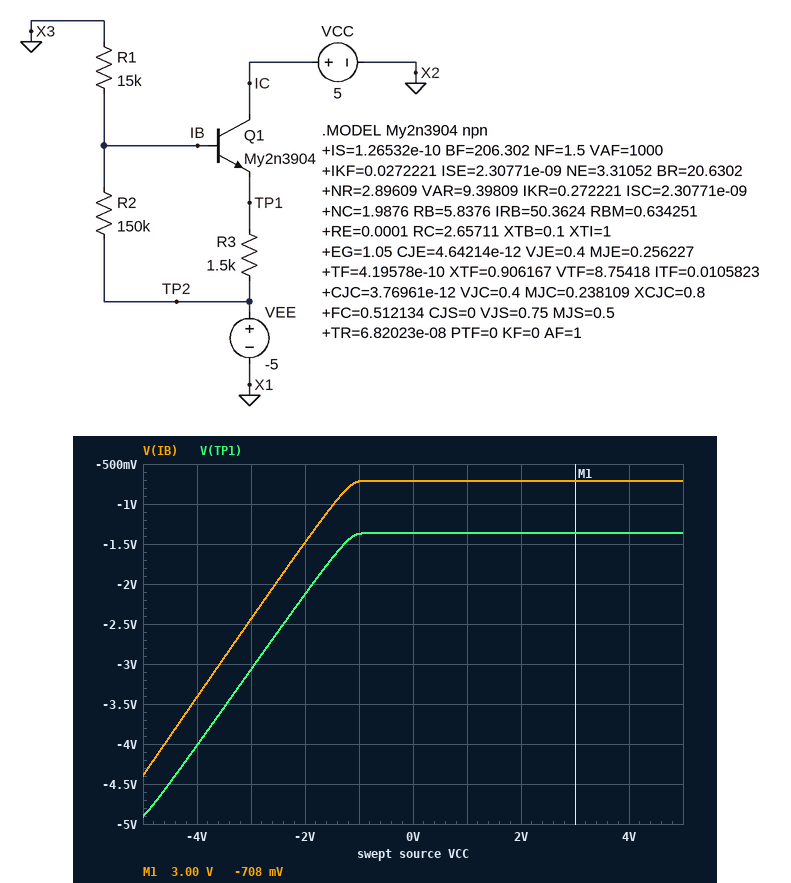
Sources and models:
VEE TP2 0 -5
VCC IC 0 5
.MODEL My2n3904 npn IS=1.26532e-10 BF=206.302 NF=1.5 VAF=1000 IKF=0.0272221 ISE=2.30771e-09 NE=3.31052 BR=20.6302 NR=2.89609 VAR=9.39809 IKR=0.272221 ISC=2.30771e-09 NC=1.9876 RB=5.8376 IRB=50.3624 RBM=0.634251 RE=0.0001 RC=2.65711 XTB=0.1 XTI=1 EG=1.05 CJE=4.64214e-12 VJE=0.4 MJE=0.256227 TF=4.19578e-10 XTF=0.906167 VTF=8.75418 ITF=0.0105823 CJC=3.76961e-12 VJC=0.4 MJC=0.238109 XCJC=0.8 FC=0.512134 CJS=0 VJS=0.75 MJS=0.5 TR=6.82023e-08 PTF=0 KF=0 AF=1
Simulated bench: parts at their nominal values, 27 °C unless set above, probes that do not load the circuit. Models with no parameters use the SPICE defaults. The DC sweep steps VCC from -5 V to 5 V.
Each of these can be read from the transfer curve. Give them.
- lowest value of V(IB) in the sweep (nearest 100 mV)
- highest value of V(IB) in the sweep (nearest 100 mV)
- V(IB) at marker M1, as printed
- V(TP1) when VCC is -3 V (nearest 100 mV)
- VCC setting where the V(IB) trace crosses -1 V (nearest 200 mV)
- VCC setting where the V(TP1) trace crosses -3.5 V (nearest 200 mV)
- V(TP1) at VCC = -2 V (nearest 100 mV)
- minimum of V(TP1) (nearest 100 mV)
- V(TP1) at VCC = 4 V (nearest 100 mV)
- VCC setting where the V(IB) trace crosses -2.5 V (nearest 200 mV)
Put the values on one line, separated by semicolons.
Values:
-4.4 V; -700 mV; -708 mV; -3.1 V; -1.4 V; -3.4 V; -2.1 V; -4.9 V; -1.4 V; -3.0 V
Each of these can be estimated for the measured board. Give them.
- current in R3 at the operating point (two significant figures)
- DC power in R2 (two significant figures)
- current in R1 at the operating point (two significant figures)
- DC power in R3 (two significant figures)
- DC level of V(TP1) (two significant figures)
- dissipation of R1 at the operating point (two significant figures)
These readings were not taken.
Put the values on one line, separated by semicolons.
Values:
2.4 mA; 120 µW; 47 µA; 8.8 mW; -1.4 V; 33 µW
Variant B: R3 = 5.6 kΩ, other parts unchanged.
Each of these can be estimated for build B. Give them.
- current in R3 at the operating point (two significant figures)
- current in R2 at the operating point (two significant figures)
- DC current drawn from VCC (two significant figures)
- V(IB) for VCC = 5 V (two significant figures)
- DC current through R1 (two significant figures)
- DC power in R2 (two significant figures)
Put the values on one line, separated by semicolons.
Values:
690 µA; 30 µA; 680 µA; -540 mV; 36 µA; 130 µW
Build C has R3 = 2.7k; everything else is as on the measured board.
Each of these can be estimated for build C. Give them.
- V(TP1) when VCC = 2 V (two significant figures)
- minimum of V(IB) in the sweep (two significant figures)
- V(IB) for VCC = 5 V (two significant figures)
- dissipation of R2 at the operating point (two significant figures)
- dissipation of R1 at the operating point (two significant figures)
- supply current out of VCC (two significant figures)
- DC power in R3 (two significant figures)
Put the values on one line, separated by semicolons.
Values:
-1.2 V; -4.4 V; -610 mV; 130 µW; 25 µW; 1.4 mA; 5.2 mW
